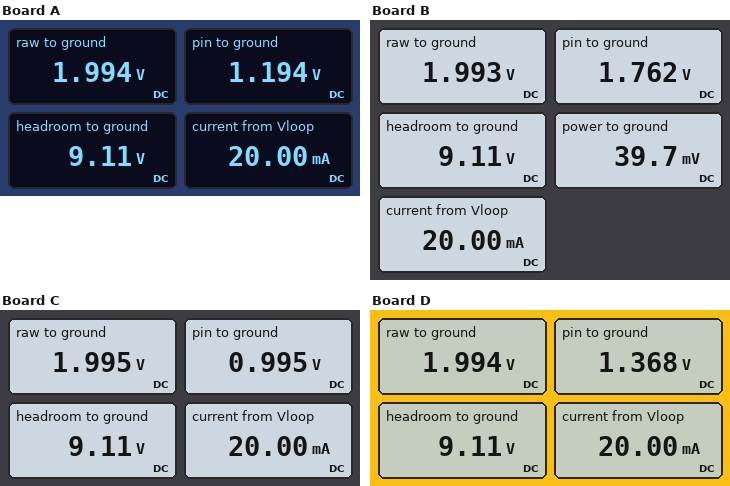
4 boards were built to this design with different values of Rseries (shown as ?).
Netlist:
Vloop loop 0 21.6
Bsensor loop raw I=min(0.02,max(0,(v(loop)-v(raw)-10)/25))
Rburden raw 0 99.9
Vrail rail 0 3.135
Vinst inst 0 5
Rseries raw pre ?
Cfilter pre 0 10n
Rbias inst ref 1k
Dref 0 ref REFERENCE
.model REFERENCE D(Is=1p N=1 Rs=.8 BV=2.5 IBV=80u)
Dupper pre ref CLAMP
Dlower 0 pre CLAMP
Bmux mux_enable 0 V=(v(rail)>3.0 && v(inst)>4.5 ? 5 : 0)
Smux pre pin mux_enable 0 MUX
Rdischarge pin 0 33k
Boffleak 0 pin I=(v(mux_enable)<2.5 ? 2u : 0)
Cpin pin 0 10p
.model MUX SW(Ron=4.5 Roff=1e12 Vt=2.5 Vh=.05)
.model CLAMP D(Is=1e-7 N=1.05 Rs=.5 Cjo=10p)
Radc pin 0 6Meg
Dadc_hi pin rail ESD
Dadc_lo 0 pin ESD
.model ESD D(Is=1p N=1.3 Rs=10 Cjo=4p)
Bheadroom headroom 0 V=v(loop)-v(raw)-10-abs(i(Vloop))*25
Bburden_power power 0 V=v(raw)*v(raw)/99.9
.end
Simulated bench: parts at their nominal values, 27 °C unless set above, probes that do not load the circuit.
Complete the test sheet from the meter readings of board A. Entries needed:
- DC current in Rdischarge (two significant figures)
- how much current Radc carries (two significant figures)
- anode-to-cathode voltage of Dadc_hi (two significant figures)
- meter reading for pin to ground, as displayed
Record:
36 µA
200 nA
-1.9 V
1.194 V
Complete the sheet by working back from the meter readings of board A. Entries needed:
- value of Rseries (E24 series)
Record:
22 kΩ
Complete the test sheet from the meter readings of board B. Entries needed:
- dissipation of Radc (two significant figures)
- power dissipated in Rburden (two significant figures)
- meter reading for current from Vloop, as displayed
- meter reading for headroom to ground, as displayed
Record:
520 nW
40 mW
20.00 mA
9.11 V
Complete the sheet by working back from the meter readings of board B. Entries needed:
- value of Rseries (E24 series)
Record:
4.3 kΩ
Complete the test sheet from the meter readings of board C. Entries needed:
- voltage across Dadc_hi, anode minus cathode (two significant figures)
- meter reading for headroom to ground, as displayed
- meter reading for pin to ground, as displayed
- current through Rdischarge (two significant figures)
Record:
-2.1 V
9.11 V
0.995 V
30 µA
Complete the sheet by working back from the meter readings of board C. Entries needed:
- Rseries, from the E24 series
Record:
33 kΩ
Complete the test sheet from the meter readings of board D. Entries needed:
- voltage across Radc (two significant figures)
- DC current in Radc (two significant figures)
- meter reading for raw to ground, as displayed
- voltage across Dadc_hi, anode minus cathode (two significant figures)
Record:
1.4 V
230 nA
1.994 V
-1.8 V
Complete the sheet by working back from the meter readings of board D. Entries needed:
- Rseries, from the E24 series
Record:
15 kΩ
